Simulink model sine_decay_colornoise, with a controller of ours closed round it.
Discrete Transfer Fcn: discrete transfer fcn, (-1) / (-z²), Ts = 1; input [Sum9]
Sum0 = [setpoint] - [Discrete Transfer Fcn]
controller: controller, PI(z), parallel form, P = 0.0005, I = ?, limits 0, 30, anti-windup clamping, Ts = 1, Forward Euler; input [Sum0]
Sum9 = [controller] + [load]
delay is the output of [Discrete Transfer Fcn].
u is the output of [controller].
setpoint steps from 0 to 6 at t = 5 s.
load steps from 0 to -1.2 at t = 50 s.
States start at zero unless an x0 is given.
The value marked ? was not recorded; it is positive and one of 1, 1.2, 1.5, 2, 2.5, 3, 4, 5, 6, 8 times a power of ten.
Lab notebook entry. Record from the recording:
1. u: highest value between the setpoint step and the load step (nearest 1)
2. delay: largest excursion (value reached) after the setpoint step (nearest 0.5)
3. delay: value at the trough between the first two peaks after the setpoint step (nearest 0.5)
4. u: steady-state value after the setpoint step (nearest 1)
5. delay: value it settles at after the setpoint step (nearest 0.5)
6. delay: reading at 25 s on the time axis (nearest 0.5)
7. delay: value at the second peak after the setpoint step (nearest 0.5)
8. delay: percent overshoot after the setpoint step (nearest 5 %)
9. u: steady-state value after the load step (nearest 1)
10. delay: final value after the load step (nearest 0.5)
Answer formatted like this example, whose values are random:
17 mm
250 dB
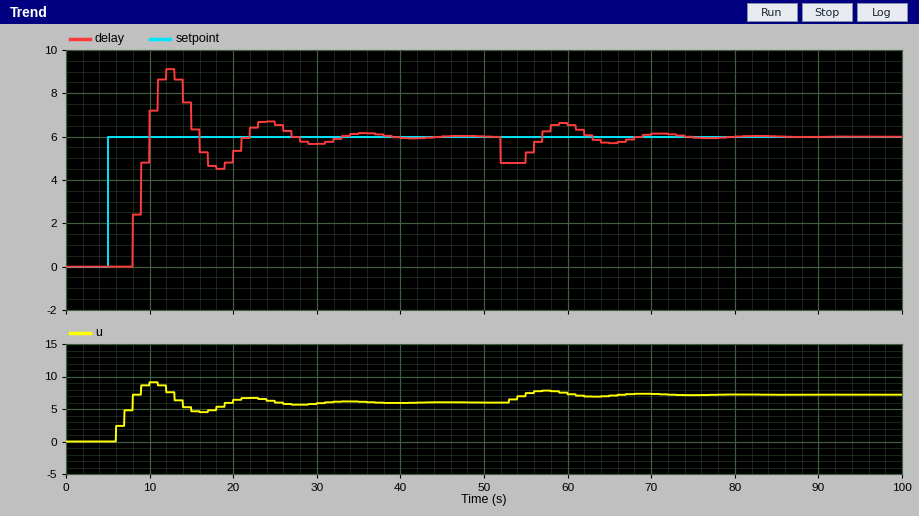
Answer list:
9
9.0
4.5
6
6.0
6.5
6.5
50 %
7
6.0
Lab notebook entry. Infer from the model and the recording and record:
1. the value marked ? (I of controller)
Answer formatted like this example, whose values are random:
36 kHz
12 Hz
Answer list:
0.4
